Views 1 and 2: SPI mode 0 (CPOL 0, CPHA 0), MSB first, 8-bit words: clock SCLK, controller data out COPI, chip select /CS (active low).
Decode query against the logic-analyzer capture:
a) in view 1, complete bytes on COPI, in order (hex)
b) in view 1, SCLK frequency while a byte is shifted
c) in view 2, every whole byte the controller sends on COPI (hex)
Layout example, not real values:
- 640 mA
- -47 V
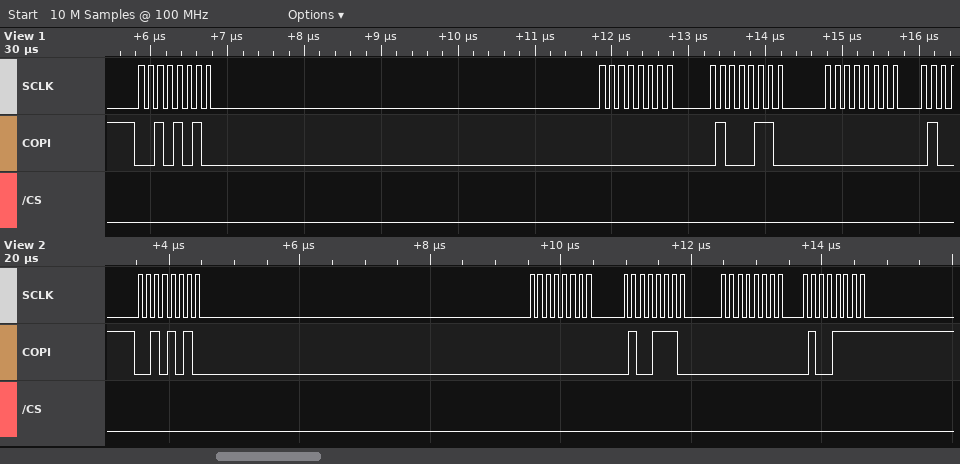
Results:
- 0x2A 0x00 0x46 0x00
- 8 MHz
- 0x2A 0x00 0x4E 0x00 0x4F
